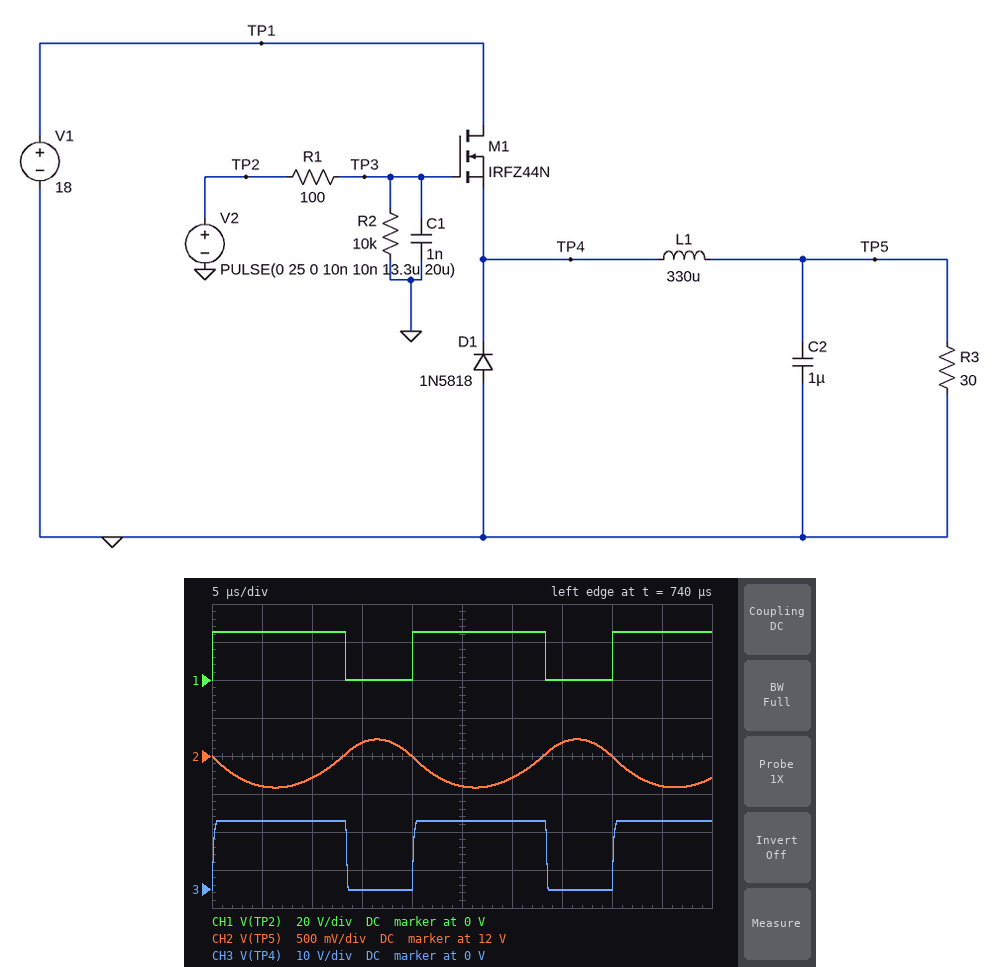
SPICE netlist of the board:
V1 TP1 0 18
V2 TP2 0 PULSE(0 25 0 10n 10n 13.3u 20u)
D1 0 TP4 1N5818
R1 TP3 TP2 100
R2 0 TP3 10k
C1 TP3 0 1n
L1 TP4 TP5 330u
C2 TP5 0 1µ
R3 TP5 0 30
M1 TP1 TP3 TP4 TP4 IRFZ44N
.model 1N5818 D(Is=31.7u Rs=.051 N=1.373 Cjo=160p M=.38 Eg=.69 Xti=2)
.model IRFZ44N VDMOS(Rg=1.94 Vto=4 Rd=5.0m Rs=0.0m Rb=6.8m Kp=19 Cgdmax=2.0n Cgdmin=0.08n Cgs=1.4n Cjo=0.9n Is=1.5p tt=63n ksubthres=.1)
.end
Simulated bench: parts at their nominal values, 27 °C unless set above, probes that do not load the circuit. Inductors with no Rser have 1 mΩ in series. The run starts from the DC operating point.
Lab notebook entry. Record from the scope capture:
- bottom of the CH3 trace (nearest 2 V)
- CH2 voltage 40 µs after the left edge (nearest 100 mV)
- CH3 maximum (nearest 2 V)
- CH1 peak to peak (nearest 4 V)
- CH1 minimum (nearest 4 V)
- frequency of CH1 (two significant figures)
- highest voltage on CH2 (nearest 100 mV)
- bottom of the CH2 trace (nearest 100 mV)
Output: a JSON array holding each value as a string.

["0 V", "12.0 V", "18 V", "24 V", "0 V", "50 kHz", "12.2 V", "11.6 V"]
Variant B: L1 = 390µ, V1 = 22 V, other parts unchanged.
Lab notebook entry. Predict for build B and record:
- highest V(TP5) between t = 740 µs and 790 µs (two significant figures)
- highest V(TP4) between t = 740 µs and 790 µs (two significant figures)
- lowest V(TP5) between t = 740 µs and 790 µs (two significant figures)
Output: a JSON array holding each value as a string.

["14 V", "21 V", "13 V"]
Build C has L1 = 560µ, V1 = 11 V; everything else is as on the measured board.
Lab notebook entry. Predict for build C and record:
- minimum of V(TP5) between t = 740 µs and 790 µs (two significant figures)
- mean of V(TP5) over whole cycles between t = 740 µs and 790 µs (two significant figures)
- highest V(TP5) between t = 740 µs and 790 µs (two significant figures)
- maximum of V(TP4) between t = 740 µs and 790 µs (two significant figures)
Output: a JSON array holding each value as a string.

["7.2 V", "7.3 V", "7.5 V", "11 V"]
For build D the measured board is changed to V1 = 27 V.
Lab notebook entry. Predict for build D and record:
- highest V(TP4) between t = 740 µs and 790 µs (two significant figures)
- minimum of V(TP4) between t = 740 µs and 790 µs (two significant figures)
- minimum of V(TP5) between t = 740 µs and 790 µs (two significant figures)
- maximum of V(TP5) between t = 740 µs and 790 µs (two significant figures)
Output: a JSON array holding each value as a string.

["21 V", "-380 mV", "13 V", "14 V"]
